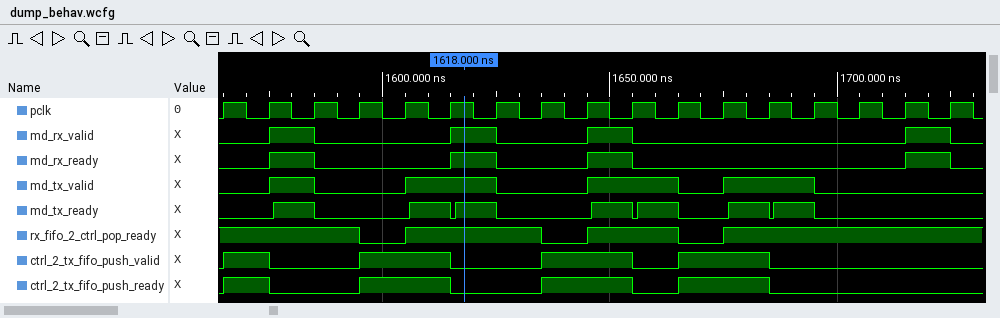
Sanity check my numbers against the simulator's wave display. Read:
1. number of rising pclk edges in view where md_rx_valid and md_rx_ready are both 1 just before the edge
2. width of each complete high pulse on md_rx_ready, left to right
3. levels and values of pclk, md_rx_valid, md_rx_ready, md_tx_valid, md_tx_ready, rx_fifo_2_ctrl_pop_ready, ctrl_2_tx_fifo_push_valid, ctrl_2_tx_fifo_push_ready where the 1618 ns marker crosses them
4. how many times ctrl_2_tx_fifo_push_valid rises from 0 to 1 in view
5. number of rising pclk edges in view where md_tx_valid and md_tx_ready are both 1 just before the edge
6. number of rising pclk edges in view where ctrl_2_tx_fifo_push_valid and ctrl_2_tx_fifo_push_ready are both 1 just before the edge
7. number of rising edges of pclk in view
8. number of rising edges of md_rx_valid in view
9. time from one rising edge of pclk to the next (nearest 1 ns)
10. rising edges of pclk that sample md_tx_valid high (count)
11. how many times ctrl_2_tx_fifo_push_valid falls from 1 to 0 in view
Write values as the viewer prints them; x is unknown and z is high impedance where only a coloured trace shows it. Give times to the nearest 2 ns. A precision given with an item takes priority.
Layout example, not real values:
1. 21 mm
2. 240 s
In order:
1. 4
2. 10 ns, 10 ns, 10 ns, 10 ns
3. pclk=1, md_rx_valid=1, md_rx_ready=1, md_tx_valid=1, md_tx_ready=1, rx_fifo_2_ctrl_pop_ready=1, ctrl_2_tx_fifo_push_valid=0, ctrl_2_tx_fifo_push_ready=0
4. 4
5. 7
6. 7
7. 17
8. 4
9. 10 ns
10. 7
11. 4
